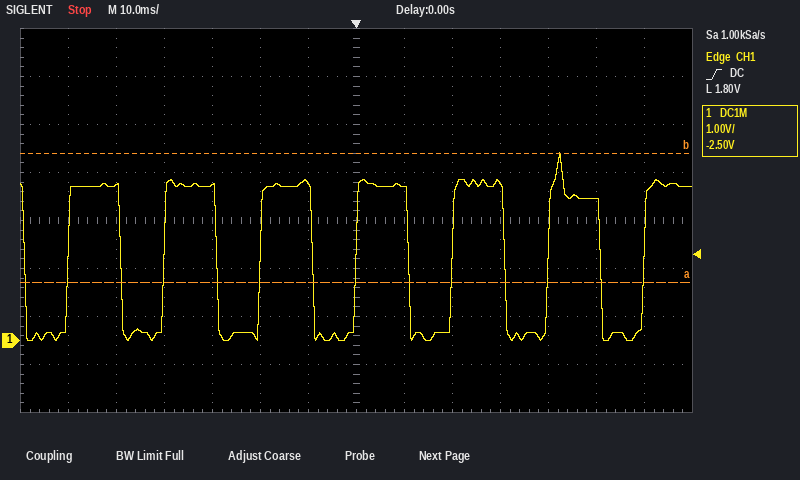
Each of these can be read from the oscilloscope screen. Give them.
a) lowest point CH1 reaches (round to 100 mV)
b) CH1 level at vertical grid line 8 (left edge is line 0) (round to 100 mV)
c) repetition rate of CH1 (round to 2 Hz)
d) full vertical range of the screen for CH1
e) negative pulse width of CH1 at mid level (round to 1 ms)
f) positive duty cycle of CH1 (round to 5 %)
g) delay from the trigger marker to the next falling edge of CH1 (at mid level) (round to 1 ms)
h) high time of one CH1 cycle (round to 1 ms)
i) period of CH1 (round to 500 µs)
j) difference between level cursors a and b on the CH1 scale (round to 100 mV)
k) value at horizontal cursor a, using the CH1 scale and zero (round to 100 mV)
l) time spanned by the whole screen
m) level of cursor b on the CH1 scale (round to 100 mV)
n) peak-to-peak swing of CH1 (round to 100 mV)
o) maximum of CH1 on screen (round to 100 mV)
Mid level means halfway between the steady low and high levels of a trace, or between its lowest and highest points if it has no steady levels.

0.0 V
3.2 V
50 Hz
8 V
9 ms
55 %
11 ms
11 ms
20.0 ms
2.7 V
1.2 V
140 ms
3.9 V
3.9 V
3.9 V
